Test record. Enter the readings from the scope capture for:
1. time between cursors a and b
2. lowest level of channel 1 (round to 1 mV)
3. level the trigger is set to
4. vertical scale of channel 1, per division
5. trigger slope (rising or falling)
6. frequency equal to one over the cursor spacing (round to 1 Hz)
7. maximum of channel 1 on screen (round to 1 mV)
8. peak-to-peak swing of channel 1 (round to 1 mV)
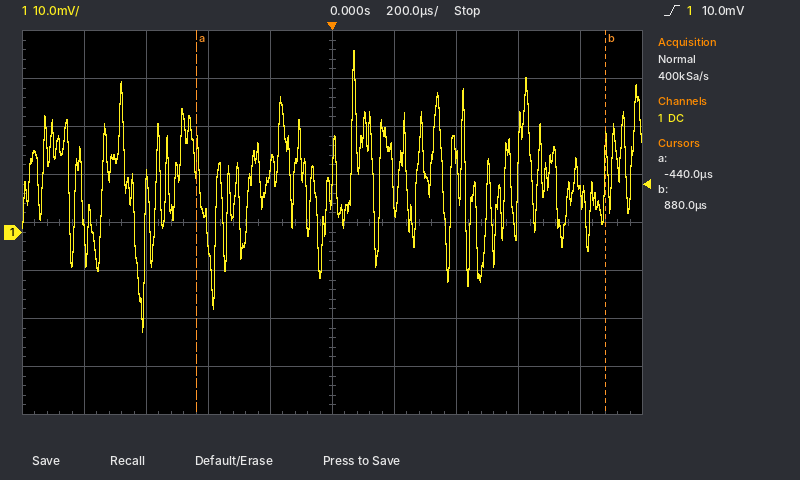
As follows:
1.32 ms
-21 mV
10.0 mV
10 mV
rising
758 Hz
38 mV
59 mV
